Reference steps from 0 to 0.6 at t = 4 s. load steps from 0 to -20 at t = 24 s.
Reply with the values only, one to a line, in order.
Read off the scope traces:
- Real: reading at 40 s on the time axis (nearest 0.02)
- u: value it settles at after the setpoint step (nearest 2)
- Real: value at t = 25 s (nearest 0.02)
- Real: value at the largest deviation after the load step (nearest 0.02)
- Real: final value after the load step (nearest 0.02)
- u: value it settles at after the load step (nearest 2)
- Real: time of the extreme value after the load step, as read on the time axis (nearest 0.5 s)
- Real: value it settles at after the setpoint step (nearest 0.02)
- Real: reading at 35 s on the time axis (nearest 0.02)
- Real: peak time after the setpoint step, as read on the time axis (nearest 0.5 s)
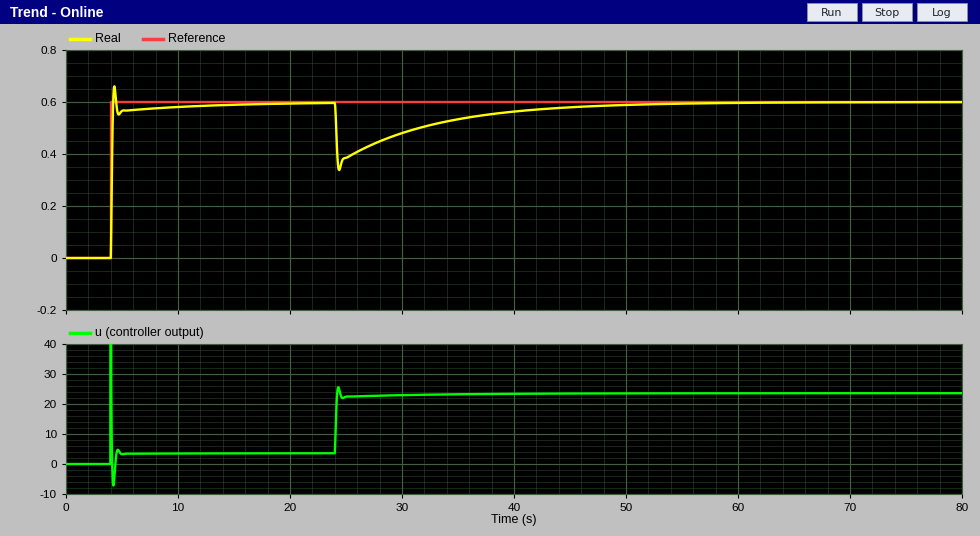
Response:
0.56
4
0.38
0.34
0.60
24
24.5 s
0.60
0.54
4.5 s
